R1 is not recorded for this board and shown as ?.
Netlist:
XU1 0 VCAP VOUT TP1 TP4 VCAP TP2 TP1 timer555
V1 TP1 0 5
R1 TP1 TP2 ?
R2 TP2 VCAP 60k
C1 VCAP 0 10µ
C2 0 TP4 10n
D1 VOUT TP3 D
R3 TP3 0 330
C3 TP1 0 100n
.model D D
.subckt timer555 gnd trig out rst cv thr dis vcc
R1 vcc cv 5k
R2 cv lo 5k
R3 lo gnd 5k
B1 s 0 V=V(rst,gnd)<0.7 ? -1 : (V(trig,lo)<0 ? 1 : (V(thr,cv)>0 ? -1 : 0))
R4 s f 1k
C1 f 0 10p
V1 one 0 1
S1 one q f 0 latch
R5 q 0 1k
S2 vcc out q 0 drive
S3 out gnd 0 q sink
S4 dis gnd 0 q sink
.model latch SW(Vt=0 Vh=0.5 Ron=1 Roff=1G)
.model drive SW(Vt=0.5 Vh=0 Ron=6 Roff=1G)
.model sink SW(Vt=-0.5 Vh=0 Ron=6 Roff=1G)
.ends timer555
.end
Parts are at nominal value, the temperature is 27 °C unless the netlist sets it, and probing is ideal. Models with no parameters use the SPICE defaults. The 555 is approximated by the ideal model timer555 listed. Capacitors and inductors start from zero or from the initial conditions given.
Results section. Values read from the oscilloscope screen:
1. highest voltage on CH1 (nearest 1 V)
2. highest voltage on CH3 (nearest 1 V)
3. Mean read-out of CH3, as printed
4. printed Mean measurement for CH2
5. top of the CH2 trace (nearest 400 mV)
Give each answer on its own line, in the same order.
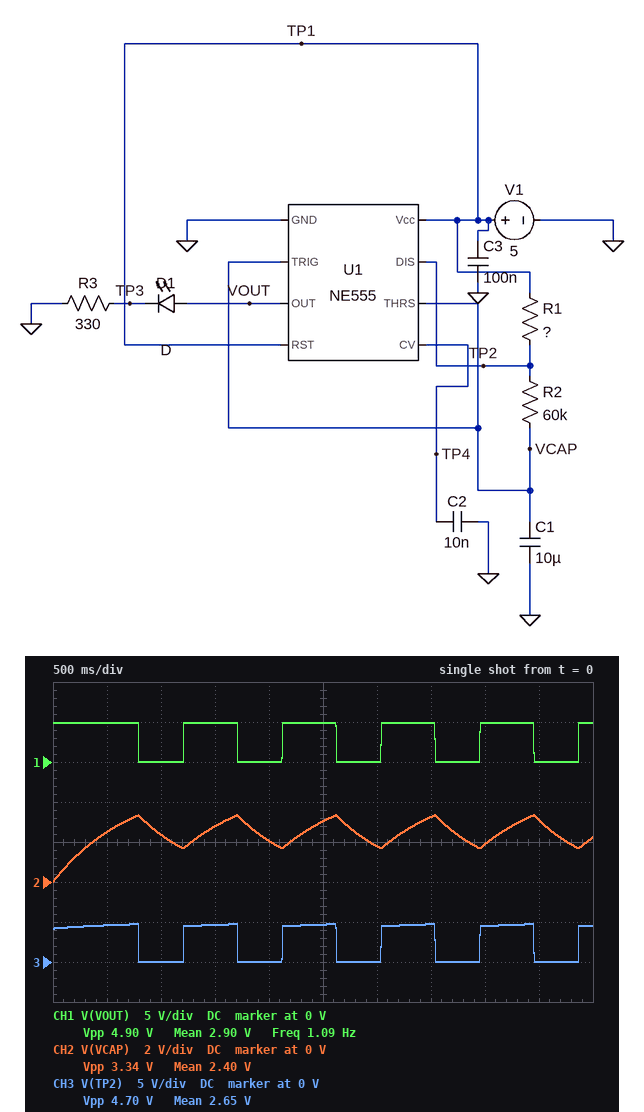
5 V
5 V
2.65 V
2.40 V
3.2 V
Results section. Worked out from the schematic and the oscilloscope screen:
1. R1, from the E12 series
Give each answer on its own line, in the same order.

12 kΩ
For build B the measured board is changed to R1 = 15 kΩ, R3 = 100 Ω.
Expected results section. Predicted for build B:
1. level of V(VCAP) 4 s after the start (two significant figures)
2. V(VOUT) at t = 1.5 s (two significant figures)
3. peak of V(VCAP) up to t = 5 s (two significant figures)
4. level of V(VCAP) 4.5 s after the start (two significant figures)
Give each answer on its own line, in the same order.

1.8 V
4.8 V
3.3 V
3.2 V
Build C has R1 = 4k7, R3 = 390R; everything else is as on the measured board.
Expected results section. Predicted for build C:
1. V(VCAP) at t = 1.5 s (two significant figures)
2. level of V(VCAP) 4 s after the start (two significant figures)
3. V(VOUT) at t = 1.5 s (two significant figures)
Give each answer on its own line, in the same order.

3.1 V
2.8 V
4.9 V
